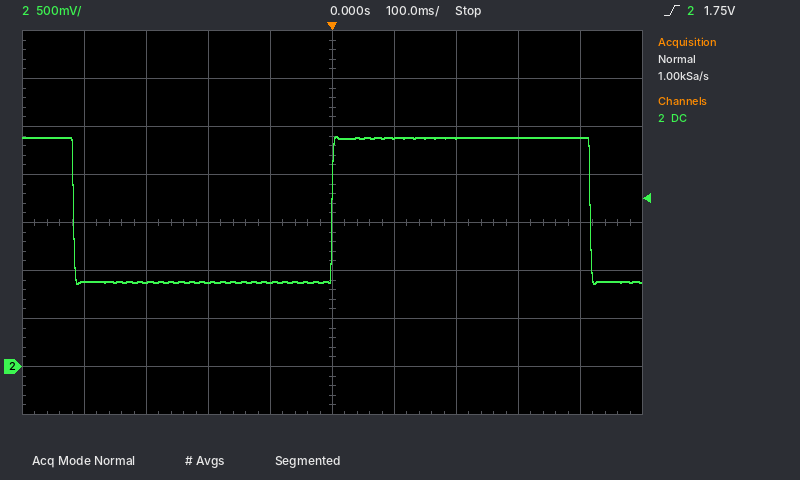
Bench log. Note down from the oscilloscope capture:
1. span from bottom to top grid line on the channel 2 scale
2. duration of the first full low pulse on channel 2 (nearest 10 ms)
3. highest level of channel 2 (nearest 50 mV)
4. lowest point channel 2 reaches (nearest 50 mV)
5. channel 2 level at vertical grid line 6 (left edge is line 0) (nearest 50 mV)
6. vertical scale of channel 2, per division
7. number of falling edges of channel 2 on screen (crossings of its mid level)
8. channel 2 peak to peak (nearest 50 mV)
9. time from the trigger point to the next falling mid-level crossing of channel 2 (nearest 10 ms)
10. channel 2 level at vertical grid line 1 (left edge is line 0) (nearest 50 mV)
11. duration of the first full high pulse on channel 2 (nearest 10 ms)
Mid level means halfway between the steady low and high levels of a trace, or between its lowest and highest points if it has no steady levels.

4 V
420 ms
2.40 V
850 mV
2.40 V
500 mV
2
1.55 V
420 ms
900 mV
420 ms
